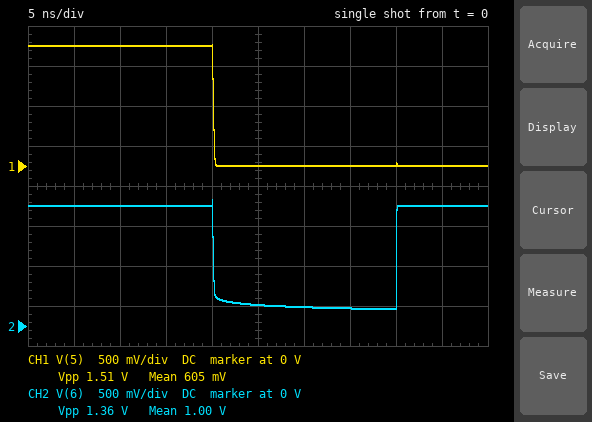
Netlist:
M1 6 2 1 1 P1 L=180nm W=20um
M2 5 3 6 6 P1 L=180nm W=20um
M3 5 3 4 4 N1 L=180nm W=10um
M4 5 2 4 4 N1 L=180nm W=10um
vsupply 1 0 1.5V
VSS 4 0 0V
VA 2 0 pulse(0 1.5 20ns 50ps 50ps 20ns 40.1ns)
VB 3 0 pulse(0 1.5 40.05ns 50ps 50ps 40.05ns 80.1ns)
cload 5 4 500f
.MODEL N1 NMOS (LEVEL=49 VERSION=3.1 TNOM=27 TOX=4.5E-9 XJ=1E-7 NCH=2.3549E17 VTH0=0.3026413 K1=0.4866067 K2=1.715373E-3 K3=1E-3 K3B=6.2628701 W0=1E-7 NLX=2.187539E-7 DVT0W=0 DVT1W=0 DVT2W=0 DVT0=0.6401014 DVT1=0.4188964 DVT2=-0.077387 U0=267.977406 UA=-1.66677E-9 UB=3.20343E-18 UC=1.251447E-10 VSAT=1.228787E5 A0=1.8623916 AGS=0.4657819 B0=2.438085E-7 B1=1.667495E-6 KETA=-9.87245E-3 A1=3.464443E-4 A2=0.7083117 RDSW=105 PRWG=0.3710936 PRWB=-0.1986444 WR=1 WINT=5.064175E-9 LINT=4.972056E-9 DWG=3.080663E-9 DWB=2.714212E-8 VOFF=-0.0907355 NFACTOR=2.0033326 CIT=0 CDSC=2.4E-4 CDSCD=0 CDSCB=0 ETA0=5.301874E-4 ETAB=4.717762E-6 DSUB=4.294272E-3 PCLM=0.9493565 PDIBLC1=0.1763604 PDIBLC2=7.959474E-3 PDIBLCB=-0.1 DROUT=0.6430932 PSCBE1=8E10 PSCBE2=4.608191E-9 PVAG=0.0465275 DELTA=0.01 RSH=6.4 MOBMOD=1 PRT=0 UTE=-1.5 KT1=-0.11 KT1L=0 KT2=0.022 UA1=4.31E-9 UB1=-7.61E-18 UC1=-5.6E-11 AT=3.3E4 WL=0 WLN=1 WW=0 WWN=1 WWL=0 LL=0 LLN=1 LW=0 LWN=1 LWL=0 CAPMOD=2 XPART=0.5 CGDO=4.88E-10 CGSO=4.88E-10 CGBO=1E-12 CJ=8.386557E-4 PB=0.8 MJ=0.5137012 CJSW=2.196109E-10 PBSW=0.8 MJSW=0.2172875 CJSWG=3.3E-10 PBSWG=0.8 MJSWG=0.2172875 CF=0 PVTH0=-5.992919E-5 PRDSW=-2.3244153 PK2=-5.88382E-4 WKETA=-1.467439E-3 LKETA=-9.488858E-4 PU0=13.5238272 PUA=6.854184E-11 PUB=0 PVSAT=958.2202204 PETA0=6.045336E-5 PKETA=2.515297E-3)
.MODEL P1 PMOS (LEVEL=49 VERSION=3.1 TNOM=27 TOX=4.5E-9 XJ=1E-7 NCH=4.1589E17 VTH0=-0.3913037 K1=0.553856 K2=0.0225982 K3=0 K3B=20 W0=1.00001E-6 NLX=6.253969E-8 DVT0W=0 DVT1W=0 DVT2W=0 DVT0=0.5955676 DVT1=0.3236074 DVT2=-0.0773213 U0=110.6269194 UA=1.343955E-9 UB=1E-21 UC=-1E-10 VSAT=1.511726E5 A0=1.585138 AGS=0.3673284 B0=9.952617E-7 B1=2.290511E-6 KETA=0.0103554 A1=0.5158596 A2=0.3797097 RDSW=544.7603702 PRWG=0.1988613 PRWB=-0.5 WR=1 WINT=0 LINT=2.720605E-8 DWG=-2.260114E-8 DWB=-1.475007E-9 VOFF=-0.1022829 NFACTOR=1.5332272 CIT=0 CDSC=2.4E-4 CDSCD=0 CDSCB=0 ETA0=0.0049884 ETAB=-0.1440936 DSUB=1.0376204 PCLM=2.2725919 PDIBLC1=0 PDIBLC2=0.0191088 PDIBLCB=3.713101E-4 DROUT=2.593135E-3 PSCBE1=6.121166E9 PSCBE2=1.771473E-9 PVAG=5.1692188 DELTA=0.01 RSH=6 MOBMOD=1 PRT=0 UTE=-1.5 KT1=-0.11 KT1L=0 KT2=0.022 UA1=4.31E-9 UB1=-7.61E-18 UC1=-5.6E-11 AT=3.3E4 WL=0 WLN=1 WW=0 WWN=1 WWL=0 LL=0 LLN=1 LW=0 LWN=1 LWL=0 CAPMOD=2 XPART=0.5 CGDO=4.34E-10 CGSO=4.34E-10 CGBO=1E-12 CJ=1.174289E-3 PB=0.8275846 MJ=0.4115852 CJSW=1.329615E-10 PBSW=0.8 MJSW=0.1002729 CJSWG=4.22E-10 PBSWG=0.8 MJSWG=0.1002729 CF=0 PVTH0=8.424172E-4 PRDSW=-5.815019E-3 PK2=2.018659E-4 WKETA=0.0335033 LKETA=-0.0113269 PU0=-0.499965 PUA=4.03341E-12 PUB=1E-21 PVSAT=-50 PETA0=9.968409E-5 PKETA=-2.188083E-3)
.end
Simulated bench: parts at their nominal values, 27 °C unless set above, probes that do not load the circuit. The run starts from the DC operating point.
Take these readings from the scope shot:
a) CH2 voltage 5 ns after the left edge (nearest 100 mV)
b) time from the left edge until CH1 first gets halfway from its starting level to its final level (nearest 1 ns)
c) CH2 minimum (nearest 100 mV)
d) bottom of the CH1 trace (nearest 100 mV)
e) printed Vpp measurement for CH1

1.5 V
20 ns
200 mV
0 V
1.51 V
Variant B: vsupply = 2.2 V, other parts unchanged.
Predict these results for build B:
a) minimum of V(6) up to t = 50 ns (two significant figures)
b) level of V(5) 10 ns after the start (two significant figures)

720 mV
2.2 V
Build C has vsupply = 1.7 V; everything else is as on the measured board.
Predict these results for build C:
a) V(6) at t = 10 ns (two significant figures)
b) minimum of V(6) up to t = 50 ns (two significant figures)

1.7 V
230 mV
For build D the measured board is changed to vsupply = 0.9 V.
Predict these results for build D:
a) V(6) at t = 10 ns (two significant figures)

900 mV
